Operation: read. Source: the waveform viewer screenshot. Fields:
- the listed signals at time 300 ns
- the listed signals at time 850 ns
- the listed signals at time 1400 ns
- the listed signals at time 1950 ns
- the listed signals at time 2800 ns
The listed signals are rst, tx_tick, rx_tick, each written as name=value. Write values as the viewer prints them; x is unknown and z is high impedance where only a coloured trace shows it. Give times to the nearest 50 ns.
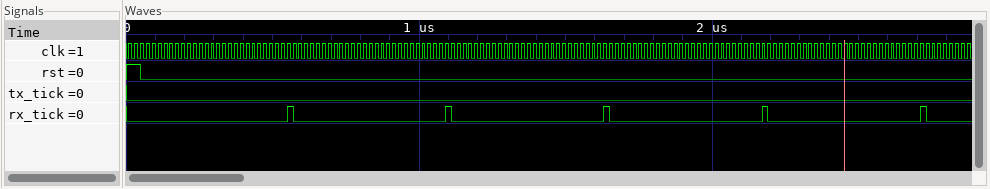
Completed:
rst=0, tx_tick=0, rx_tick=0
rst=0, tx_tick=0, rx_tick=0
rst=0, tx_tick=0, rx_tick=0
rst=0, tx_tick=0, rx_tick=0
rst=0, tx_tick=0, rx_tick=0
